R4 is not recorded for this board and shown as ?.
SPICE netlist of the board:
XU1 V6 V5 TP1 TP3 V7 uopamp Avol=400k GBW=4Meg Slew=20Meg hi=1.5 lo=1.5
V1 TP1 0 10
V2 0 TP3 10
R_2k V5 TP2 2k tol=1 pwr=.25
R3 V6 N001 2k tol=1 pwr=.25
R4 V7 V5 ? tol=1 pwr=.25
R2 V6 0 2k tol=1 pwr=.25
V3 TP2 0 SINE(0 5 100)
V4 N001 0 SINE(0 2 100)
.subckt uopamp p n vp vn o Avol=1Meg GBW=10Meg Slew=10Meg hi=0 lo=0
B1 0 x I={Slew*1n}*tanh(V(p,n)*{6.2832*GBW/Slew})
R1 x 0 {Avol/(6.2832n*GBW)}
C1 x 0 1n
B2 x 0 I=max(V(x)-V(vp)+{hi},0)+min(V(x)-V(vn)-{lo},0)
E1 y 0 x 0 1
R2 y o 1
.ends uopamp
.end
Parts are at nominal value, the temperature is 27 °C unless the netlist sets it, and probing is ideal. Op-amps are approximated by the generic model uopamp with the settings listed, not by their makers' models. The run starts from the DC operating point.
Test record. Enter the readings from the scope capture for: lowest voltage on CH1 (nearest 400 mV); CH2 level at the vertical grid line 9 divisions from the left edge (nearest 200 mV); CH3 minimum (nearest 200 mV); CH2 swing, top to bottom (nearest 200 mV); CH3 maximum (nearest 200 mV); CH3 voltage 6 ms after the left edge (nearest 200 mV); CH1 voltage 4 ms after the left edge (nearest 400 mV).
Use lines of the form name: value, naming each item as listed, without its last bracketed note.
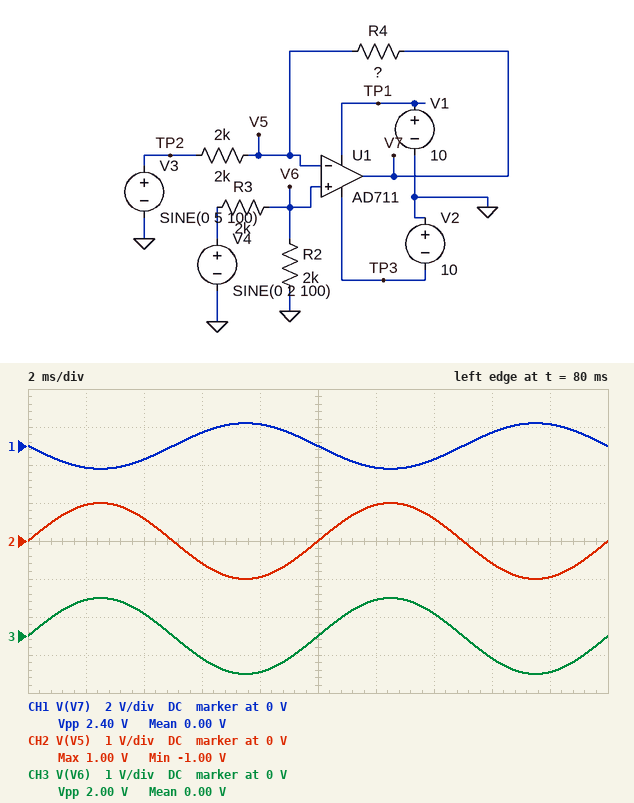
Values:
lowest voltage on CH1: -1.2 V
CH2 level at the vertical grid line 9 divisions from the left edge: -1.0 V
CH3 minimum: -1.0 V
CH2 swing, top to bottom: 2.0 V
CH3 maximum: 1.0 V
CH3 voltage 6 ms after the left edge: -600 mV
CH1 voltage 4 ms after the left edge: -800 mV
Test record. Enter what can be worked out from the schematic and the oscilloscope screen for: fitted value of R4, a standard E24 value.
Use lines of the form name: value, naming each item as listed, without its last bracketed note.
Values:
fitted value of R4, a standard E24 value: 1.1 kΩ
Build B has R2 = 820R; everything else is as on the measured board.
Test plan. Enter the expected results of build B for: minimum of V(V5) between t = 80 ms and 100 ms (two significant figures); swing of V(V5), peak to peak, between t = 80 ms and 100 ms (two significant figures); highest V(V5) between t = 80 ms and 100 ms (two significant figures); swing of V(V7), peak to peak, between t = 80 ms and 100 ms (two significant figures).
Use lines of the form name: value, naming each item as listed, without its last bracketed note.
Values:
minimum of V(V5) between t = 80 ms and 100 ms: -580 mV
swing of V(V5), peak to peak, between t = 80 ms and 100 ms: 1.2 V
highest V(V5) between t = 80 ms and 100 ms: 580 mV
swing of V(V7), peak to peak, between t = 80 ms and 100 ms: 3.7 V
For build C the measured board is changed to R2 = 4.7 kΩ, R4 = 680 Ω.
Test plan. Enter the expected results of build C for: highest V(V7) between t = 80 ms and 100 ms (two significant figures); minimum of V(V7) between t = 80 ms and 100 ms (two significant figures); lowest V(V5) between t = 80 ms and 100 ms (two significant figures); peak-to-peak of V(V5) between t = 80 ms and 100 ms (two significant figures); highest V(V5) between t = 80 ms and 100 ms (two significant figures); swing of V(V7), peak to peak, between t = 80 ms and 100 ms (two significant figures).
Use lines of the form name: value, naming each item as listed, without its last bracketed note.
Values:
highest V(V7) between t = 80 ms and 100 ms: 180 mV
minimum of V(V7) between t = 80 ms and 100 ms: -180 mV
lowest V(V5) between t = 80 ms and 100 ms: -1.4 V
peak-to-peak of V(V5) between t = 80 ms and 100 ms: 2.8 V
highest V(V5) between t = 80 ms and 100 ms: 1.4 V
swing of V(V7), peak to peak, between t = 80 ms and 100 ms: 360 mV
